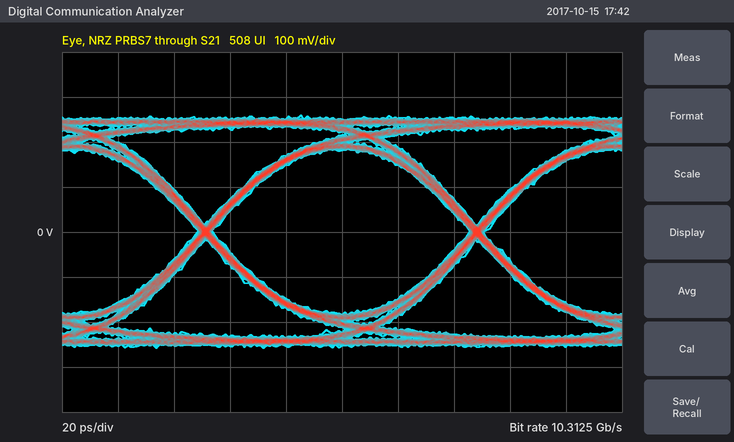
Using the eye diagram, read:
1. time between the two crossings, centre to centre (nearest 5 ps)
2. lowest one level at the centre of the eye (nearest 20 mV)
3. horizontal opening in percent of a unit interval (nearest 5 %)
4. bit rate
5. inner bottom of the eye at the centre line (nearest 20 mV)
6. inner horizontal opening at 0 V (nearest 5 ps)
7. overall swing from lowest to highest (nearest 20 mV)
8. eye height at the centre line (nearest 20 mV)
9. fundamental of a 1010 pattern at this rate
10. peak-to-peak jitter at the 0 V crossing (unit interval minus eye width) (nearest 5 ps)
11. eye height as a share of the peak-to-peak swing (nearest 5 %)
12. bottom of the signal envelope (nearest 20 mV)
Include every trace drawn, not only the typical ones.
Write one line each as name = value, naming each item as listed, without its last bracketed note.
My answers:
time between the two crossings, centre to centre = 95 ps
lowest one level at the centre of the eye = 180 mV
horizontal opening in percent of a unit interval = 95 %
bit rate = 10.3125 Gb/s
inner bottom of the eye at the centre line = -180 mV
inner horizontal opening at 0 V = 90 ps
overall swing from lowest to highest = 520 mV
eye height at the centre line = 360 mV
fundamental of a 1010 pattern at this rate = 5.15625 GHz
peak-to-peak jitter at the 0 V crossing (unit interval minus eye width) = 5 ps
eye height as a share of the peak-to-peak swing = 70 %
bottom of the signal envelope = -260 mV
